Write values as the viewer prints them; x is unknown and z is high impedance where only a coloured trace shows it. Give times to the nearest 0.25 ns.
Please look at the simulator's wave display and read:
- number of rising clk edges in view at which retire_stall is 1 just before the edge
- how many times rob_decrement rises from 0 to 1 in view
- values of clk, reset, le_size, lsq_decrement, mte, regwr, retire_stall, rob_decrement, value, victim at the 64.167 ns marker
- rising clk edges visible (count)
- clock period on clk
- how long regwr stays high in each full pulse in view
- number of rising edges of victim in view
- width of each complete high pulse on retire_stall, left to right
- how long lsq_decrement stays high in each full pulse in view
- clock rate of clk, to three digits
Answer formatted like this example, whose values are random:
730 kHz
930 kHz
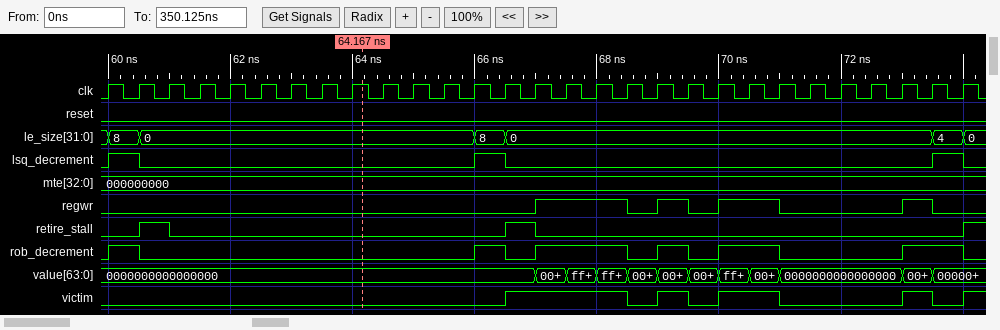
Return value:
2
6
clk=1, reset=0, le_size=0, lsq_decrement=0, mte=000000000, regwr=0, retire_stall=0, rob_decrement=0, value=0000000000000000, victim=0
29
0.5 ns
1.5 ns, 0.5 ns, 1 ns, 0.5 ns
5
0.5 ns, 0.5 ns
0.5 ns, 0.5 ns, 0.5 ns
2.00 GHz
